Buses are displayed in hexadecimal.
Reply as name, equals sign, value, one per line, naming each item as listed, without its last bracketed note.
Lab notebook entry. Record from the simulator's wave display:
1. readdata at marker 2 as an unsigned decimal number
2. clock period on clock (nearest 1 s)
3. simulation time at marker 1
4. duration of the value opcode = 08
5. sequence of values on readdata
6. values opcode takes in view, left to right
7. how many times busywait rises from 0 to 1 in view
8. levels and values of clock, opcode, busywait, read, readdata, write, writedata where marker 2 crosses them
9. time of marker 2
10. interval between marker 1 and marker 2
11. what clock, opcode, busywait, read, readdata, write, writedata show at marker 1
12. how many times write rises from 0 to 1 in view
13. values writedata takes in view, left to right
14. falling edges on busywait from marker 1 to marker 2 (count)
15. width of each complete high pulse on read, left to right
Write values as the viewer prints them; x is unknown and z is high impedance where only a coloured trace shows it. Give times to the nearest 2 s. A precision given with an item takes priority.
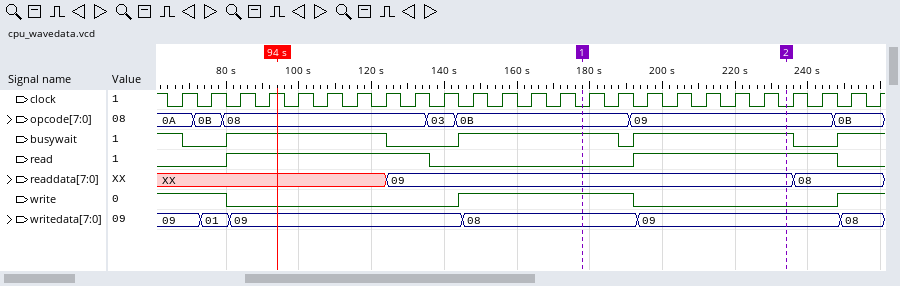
readdata at marker 2 as an unsigned decimal number = 9
clock period on clock = 8 s
simulation time at marker 1 = 178 s
duration of the value opcode = 08 = 56 s
sequence of values on readdata = XX, 09, 08
values opcode takes in view, left to right = 0A, 0B, 08, 03, 0B, 09, 0B
how many times busywait rises from 0 to 1 in view = 4
levels and values of clock, opcode, busywait, read, readdata, write, writedata where marker 2 crosses them = clock=0, opcode=09, busywait=1, read=1, readdata=09, write=0, writedata=09
time of marker 2 = 234 s
interval between marker 1 and marker 2 = 56 s
what clock, opcode, busywait, read, readdata, write, writedata show at marker 1 = clock=0, opcode=0B, busywait=1, read=0, readdata=09, write=1, writedata=08
how many times write rises from 0 to 1 in view = 2
values writedata takes in view, left to right = 09, 01, 09, 08, 09, 08
falling edges on busywait from marker 1 to marker 2 = 1
width of each complete high pulse on read, left to right = 56 s, 56 s
